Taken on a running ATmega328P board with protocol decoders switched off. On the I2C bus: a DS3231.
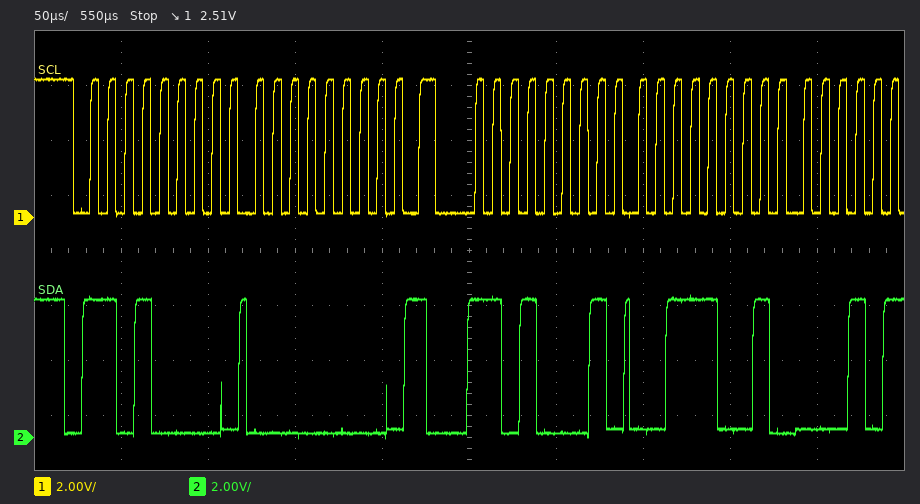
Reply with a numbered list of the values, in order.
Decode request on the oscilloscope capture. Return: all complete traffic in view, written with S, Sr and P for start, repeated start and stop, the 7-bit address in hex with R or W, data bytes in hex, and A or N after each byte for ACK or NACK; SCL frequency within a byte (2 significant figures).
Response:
1. S 68W A 00 A Sr 68R A 39 A
2. 100 kHz
